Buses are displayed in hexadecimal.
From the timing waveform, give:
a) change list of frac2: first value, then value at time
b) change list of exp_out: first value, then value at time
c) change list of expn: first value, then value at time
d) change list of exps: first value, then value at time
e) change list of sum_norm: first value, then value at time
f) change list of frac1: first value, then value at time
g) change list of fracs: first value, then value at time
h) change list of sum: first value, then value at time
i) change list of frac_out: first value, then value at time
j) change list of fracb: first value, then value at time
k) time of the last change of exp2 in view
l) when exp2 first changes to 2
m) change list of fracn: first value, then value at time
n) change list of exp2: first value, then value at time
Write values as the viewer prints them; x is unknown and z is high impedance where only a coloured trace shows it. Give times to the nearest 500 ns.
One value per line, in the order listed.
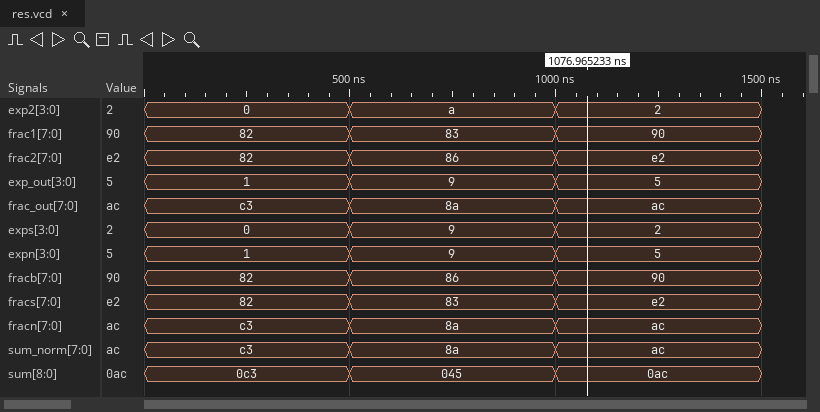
82, 86 at 500 ns, e2 at 1000 ns
1, 9 at 500 ns, 5 at 1000 ns
1, 9 at 500 ns, 5 at 1000 ns
0, 9 at 500 ns, 2 at 1000 ns
c3, 8a at 500 ns, ac at 1000 ns
82, 83 at 500 ns, 90 at 1000 ns
82, 83 at 500 ns, e2 at 1000 ns
0c3, 045 at 500 ns, 0ac at 1000 ns
c3, 8a at 500 ns, ac at 1000 ns
82, 86 at 500 ns, 90 at 1000 ns
1000 ns
1000 ns
c3, 8a at 500 ns, ac at 1000 ns
0, a at 500 ns, 2 at 1000 ns
